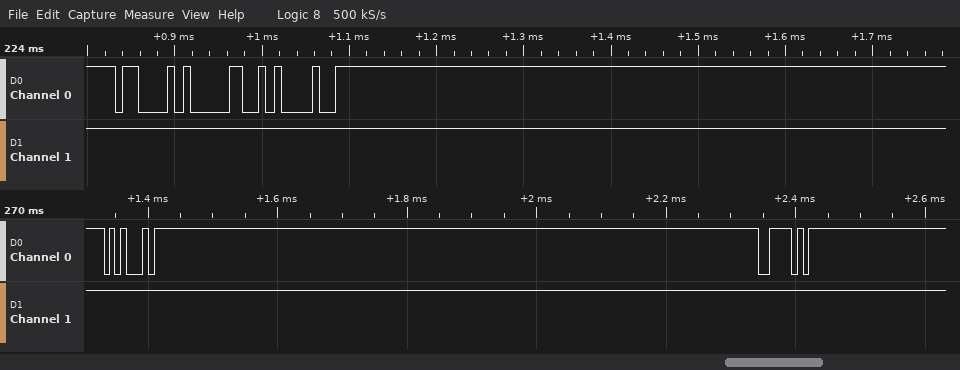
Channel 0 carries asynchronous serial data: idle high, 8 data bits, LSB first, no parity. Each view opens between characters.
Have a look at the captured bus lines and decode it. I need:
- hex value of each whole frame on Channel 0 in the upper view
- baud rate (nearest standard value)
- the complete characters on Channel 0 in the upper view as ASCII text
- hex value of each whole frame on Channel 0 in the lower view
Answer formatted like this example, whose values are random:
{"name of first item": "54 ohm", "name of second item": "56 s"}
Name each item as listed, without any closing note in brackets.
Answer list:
{"hex value of each whole frame on Channel 0 in the upper view": "43, 30, 21", "baud rate": "115200 baud", "the complete characters on Channel 0 in the upper view as ASCII text": "\"C0!\"", "hex value of each whole frame on Channel 0 in the lower view": "45, 5E"}
